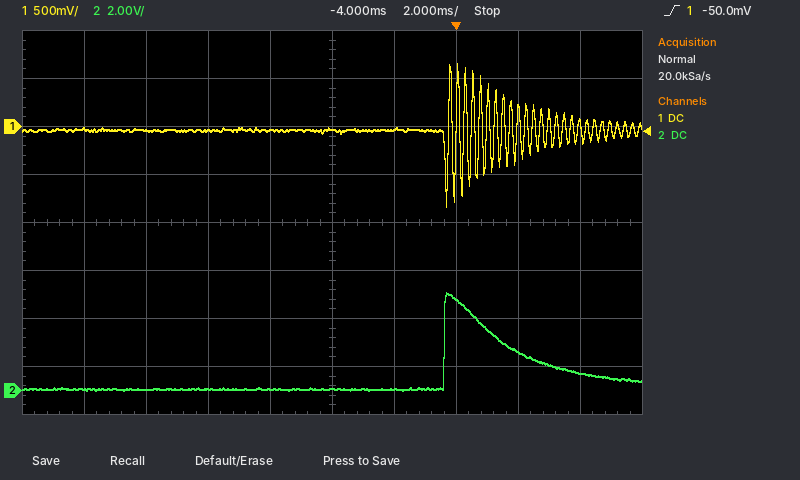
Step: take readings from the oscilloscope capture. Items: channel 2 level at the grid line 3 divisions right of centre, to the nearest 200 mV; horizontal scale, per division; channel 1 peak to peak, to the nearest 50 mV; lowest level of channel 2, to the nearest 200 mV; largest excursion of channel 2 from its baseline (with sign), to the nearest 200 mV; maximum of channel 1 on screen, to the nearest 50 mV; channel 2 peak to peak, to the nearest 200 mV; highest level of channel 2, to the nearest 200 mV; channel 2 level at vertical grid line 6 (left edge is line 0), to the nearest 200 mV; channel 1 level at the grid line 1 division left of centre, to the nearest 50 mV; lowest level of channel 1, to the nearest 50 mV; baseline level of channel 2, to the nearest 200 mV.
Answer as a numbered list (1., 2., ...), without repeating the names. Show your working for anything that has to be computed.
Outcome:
1. 1.6 V
2. 2 ms
3. 650 mV − (-850 mV) = 1.50 V
4. 0.0 V
5. 4.0 V − (0.0 V) = +4.0 V
6. 650 mV
7. 4.0 V − (0.0 V) = 4.0 V
8. 4.0 V
9. 0.0 V
10. -50 mV
11. -850 mV
12. 0.0 V
